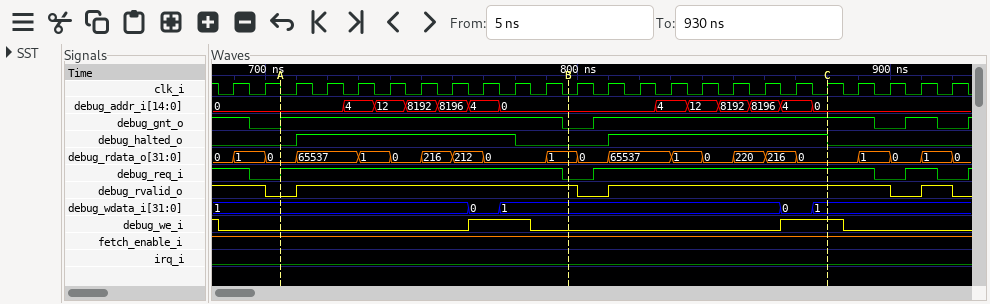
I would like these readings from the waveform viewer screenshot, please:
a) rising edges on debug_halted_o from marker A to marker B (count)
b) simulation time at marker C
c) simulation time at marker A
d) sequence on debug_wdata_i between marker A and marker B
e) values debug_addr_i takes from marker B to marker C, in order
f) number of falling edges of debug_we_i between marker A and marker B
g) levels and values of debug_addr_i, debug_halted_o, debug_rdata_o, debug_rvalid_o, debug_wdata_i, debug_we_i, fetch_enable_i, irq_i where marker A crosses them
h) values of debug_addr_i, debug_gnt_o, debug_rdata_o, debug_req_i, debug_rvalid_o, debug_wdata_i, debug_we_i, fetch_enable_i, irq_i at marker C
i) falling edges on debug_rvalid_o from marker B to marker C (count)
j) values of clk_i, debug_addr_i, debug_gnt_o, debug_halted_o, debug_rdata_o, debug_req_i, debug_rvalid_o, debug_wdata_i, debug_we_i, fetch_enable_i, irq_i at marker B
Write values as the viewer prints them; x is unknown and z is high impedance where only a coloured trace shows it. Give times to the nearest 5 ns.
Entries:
1
880 ns
705 ns
1, 0, 1
0, 4, 12, 8192, 8196, 4, 0
1
debug_addr_i=0, debug_halted_o=0, debug_rdata_o=0, debug_rvalid_o=0, debug_wdata_i=1, debug_we_i=0, fetch_enable_i=1, irq_i=0
debug_addr_i=0, debug_gnt_o=1, debug_rdata_o=0, debug_req_i=1, debug_rvalid_o=1, debug_wdata_i=1, debug_we_i=1, fetch_enable_i=1, irq_i=0
1
clk_i=0, debug_addr_i=0, debug_gnt_o=0, debug_halted_o=0, debug_rdata_o=1, debug_req_i=0, debug_rvalid_o=1, debug_wdata_i=1, debug_we_i=0, fetch_enable_i=1, irq_i=0
